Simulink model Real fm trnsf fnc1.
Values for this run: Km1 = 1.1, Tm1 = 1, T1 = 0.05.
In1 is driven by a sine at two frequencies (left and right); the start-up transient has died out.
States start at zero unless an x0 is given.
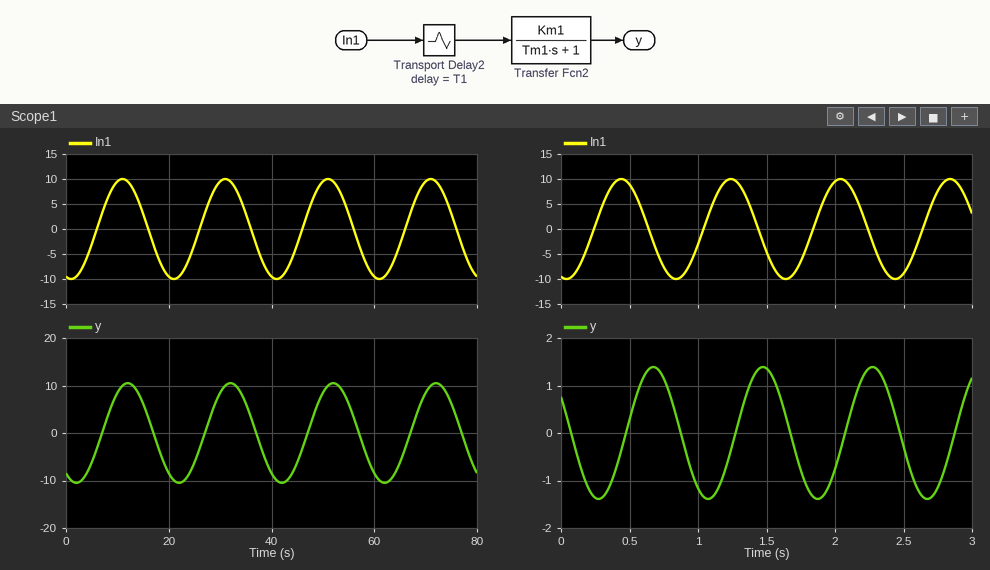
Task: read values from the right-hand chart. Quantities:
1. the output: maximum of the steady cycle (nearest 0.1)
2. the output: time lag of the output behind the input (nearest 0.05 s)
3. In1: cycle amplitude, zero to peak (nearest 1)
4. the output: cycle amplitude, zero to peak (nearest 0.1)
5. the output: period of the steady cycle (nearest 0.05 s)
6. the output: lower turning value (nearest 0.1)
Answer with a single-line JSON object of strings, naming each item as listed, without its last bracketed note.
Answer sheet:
{"the output: maximum of the steady cycle": "1.4", "the output: time lag of the output behind the input": "0.25 s", "In1: cycle amplitude, zero to peak": "10", "the output: cycle amplitude, zero to peak": "1.4", "the output: period of the steady cycle": "0.80 s", "the output: lower turning value": "-1.4"}
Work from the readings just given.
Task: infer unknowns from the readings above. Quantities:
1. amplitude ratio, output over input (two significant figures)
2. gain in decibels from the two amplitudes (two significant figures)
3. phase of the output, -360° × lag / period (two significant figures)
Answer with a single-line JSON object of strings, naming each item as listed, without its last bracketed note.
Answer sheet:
{"amplitude ratio, output over input": "0.14", "gain in decibels from the two amplitudes": "-17 dB", "phase of the output, -360° × lag / period": "-110°"}
